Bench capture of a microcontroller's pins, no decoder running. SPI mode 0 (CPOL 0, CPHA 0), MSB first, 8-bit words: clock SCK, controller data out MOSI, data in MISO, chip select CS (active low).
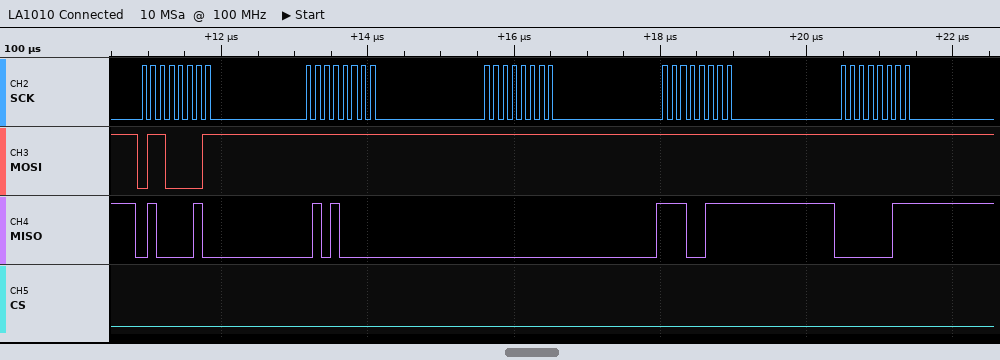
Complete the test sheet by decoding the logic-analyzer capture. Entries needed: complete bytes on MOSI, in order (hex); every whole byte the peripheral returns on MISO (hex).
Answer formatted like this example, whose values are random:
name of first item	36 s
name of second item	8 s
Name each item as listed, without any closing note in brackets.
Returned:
complete bytes on MOSI, in order	0x61 0xFF 0xFF 0xFF 0xFF
every whole byte the peripheral returns on MISO	0x42 0x50 0x00 0xE7 0x03
